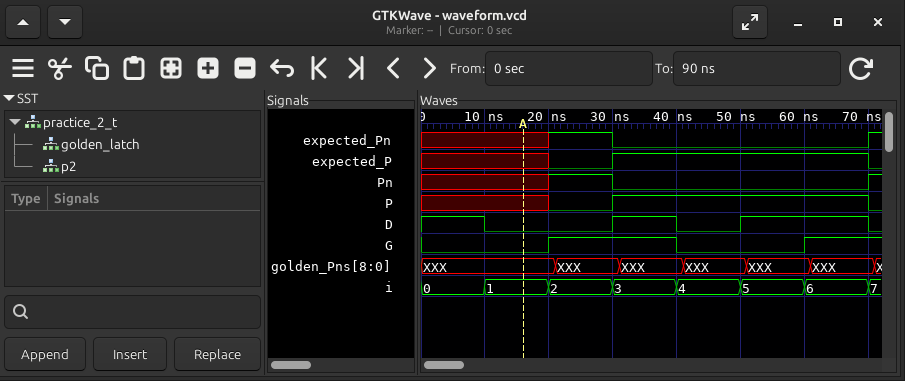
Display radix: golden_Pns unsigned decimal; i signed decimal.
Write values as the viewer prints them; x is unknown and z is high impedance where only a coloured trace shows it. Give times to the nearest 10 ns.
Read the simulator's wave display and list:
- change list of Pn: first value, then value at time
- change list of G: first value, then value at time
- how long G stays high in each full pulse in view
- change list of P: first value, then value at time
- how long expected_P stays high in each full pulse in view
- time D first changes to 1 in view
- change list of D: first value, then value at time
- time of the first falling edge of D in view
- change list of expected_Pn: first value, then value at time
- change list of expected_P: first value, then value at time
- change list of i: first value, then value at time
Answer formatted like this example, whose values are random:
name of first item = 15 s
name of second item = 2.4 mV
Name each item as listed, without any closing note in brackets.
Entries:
change list of Pn: first value, then value at time = x, 1 at 20 ns, 0 at 30 ns, 1 at 70 ns
change list of G: first value, then value at time = 0, 1 at 20 ns, 0 at 40 ns, 1 at 60 ns
how long G stays high in each full pulse in view = 20 ns
change list of P: first value, then value at time = x, 0 at 20 ns, 1 at 30 ns, 0 at 70 ns
how long expected_P stays high in each full pulse in view = 40 ns
time D first changes to 1 in view = 30 ns
change list of D: first value, then value at time = 1, 0 at 10 ns, 1 at 30 ns, 0 at 40 ns, 1 at 50 ns, 0 at 70 ns
time of the first falling edge of D in view = 10 ns
change list of expected_Pn: first value, then value at time = x, 1 at 20 ns, 0 at 30 ns, 1 at 70 ns
change list of expected_P: first value, then value at time = x, 0 at 20 ns, 1 at 30 ns, 0 at 70 ns
change list of i: first value, then value at time = 0, 1 at 10 ns, 2 at 20 ns, 3 at 30 ns, 4 at 40 ns, 5 at 50 ns, 6 at 60 ns, 7 at 70 ns
